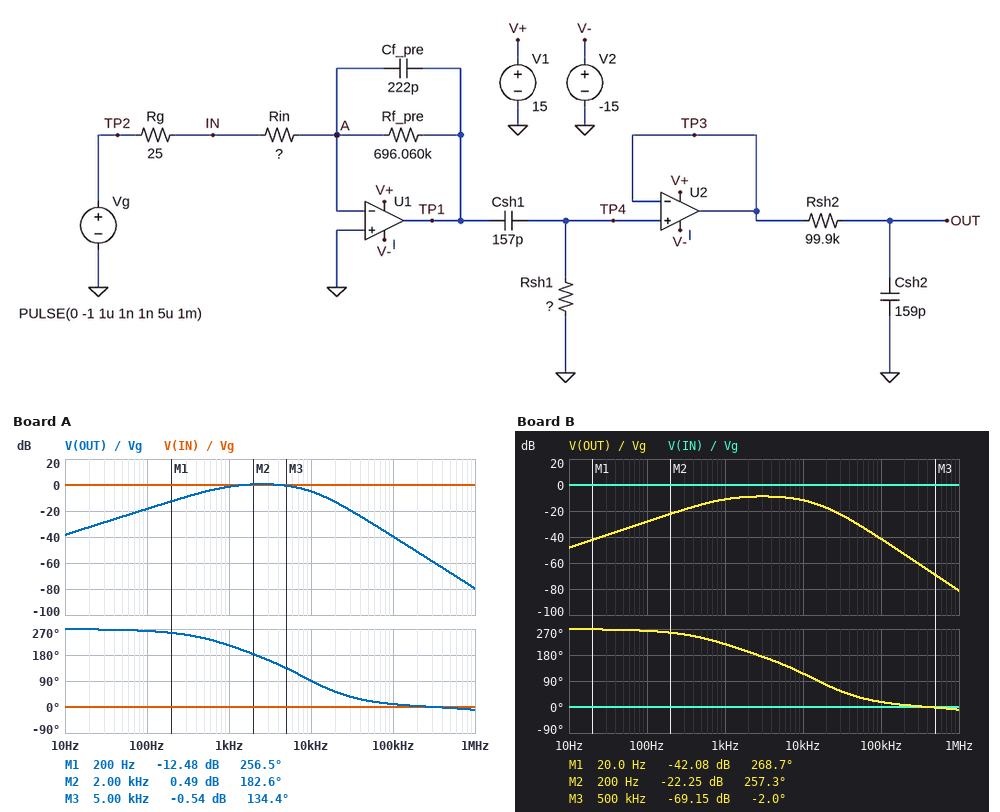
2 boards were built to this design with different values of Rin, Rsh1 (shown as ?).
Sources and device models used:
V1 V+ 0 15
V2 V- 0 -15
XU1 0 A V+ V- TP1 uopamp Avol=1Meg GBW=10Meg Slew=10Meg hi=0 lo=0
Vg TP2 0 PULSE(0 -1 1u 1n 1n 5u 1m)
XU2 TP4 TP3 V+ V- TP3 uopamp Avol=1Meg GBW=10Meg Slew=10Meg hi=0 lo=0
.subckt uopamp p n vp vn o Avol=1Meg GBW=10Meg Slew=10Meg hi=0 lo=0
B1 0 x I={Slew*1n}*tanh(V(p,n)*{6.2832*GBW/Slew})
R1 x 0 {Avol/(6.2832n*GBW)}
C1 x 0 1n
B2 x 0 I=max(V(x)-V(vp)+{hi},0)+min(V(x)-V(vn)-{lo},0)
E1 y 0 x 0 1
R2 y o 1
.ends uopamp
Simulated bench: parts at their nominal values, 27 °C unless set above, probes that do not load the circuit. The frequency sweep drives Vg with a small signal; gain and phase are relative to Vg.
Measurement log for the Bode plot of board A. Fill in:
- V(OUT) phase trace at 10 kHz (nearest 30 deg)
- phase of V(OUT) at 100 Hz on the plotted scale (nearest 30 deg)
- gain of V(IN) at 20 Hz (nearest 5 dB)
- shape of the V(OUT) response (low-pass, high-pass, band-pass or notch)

90 deg
270 deg
0 dB
band-pass
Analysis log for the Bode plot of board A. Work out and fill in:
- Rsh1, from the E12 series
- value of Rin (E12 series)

120 kΩ
68 kΩ
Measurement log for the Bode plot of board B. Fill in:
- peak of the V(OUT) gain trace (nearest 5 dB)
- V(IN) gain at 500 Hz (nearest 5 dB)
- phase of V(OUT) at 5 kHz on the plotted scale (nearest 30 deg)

-10 dB
0 dB
150 deg
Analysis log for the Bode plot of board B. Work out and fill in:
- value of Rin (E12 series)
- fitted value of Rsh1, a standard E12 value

82 kΩ
47 kΩ
